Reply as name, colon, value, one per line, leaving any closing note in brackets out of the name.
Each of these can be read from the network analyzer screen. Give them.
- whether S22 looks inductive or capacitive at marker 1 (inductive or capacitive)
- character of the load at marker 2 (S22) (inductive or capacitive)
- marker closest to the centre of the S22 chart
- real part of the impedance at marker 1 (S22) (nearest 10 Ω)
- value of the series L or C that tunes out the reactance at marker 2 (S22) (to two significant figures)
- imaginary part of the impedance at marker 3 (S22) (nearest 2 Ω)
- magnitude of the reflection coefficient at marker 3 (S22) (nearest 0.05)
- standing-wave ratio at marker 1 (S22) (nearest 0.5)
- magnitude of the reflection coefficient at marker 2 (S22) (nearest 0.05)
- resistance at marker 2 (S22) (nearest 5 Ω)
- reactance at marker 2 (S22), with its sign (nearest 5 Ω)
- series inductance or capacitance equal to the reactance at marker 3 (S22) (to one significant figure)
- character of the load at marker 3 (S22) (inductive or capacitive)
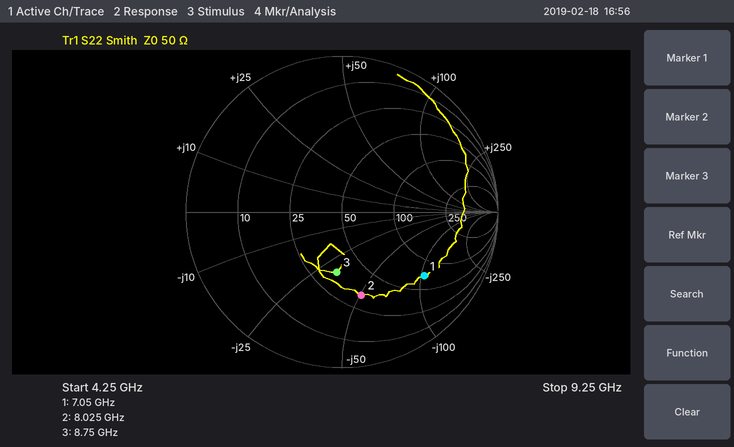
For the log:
whether S22 looks inductive or capacitive at marker 1: capacitive
character of the load at marker 2 (S22): capacitive
marker closest to the centre of the S22 chart: marker 3
real part of the impedance at marker 1 (S22): 70 Ω
value of the series L or C that tunes out the reactance at marker 2 (S22): 1.0 nH
imaginary part of the impedance at marker 3 (S22): -32 Ω
magnitude of the reflection coefficient at marker 3 (S22): 0.40
standing-wave ratio at marker 1 (S22): 5.0
magnitude of the reflection coefficient at marker 2 (S22): 0.55
resistance at marker 2 (S22): 35 Ω
reactance at marker 2 (S22), with its sign: -50 Ω
series inductance or capacitance equal to the reactance at marker 3 (S22): 600 fF
character of the load at marker 3 (S22): capacitive
